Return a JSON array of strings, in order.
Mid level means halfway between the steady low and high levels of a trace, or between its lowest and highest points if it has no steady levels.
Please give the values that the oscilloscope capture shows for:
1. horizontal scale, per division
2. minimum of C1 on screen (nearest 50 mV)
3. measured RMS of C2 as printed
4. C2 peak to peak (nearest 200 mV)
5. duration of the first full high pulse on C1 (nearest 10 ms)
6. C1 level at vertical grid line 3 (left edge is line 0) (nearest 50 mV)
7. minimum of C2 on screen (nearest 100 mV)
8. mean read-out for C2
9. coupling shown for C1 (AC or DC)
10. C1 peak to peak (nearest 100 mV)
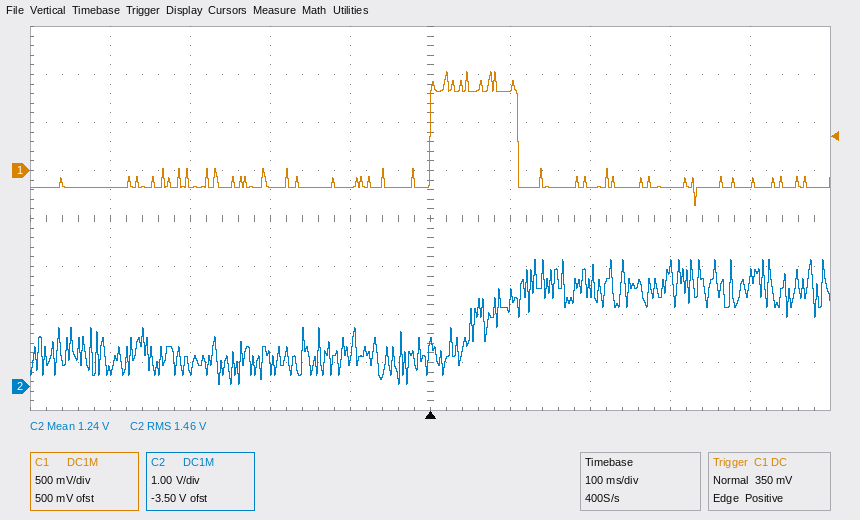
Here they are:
["100 ms", "-350 mV", "1.46 V", "2.6 V", "110 ms", "-150 mV", "0.0 V", "1.24 V", "DC", "1.40 V"]
